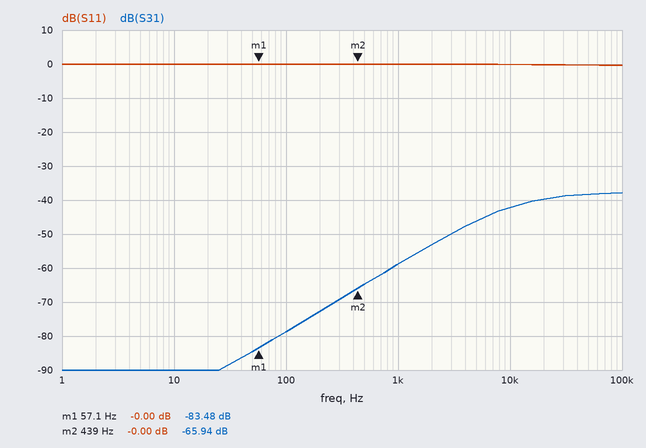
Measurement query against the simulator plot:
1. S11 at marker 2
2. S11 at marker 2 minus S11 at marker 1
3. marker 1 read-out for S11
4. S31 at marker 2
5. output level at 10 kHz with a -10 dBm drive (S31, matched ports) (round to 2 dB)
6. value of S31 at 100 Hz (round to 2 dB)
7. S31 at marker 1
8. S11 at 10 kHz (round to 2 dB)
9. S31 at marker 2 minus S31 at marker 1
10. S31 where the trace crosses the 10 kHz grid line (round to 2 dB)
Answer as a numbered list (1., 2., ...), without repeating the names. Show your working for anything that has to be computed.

1. -0.00 dB
2. -0 − (-0) = 0.00 dB
3. -0.00 dB
4. -65.94 dB
5. -10 dBm + (-42 dB) = -52 dBm
6. -78 dB
7. -83.48 dB
8. 0 dB
9. -65.94 − (-83.48) = 17.54 dB
10. -42 dB
